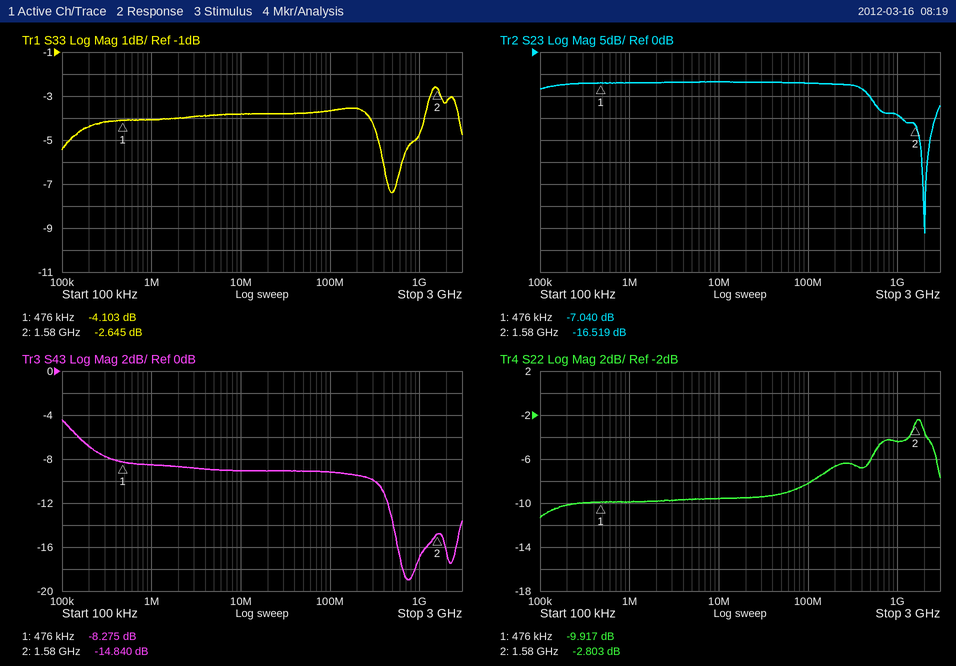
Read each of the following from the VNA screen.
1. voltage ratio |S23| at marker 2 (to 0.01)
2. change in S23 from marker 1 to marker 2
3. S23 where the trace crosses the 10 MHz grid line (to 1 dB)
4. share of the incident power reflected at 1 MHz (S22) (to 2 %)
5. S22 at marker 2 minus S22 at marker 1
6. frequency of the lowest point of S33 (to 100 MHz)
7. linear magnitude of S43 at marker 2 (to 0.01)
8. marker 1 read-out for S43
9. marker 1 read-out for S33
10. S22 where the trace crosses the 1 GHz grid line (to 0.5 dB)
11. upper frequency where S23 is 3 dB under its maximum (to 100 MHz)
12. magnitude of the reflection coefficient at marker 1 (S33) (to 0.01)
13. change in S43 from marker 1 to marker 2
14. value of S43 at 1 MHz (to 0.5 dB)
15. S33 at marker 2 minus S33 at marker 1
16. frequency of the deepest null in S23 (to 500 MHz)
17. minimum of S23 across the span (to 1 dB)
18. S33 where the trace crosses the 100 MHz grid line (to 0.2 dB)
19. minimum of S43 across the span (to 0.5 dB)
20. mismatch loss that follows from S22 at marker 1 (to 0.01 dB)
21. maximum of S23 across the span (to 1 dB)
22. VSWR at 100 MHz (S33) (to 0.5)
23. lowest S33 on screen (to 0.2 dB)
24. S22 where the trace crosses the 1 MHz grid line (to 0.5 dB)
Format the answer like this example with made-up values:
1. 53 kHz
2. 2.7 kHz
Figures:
1. 0.15
2. -9.479 dB
3. -7 dB
4. 10 %
5. 7.114 dB
6. 500 MHz
7. 0.18
8. -8.275 dB
9. -4.103 dB
10. -4.5 dB
11. 500 MHz
12. 0.62
13. -6.565 dB
14. -8.5 dB
15. 1.458 dB
16. 2.0 GHz
17. -41 dB
18. -3.6 dB
19. -19.0 dB
20. 0.47 dB
21. -7 dB
22. 5.0
23. -7.4 dB
24. -10.0 dB
